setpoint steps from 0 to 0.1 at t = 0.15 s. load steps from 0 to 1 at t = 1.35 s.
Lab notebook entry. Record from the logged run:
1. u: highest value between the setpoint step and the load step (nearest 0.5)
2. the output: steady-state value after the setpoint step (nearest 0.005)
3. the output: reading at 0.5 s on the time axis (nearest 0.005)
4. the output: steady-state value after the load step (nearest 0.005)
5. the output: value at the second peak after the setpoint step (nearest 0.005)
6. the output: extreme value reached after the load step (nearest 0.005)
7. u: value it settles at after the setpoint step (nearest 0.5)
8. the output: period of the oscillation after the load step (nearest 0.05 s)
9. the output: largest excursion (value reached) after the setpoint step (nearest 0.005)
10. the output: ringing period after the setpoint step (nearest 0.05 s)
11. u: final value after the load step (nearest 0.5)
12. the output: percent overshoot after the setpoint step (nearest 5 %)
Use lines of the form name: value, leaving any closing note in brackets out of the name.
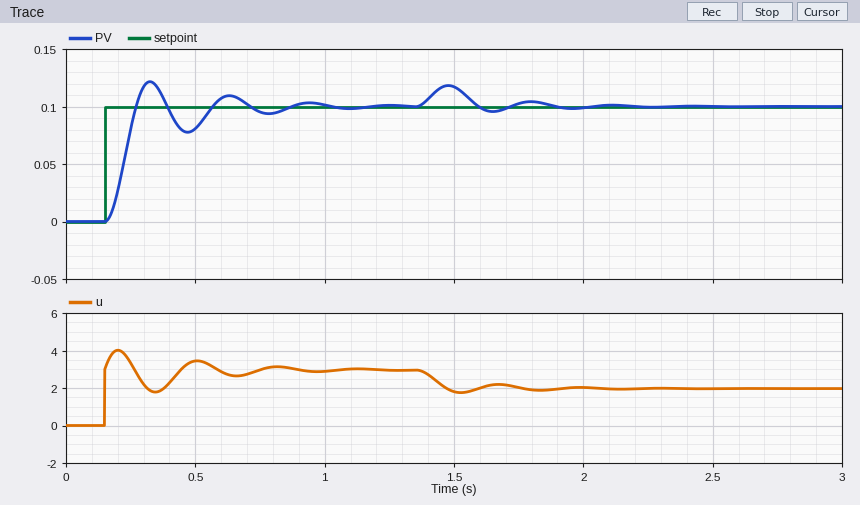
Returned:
u: highest value between the setpoint step and the load step: 4.0
the output: steady-state value after the setpoint step: 0.100
the output: reading at 0.5 s on the time axis: 0.080
the output: steady-state value after the load step: 0.100
the output: value at the second peak after the setpoint step: 0.110
the output: extreme value reached after the load step: 0.120
u: value it settles at after the setpoint step: 3.0
the output: period of the oscillation after the load step: 0.30 s
the output: largest excursion (value reached) after the setpoint step: 0.120
the output: ringing period after the setpoint step: 0.30 s
u: final value after the load step: 2.0
the output: percent overshoot after the setpoint step: 20 %
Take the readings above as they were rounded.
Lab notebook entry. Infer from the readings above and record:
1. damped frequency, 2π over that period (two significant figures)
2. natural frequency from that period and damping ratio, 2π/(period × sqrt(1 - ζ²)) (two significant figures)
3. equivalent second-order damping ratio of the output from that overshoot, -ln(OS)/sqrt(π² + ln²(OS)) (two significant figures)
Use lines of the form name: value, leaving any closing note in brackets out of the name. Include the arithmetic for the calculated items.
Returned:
damped frequency, 2π over that period: 2π / 0.3 = 21 rad/s
natural frequency from that period and damping ratio, 2π/(period × sqrt(1 - ζ²)): 2π / (0.3 × sqrt(1 - 0.46²)) = 24 rad/s
equivalent second-order damping ratio of the output from that overshoot, -ln(OS)/sqrt(π² + ln²(OS)): ln(0.2) = -1.609; 1.609 / sqrt(9.870 + 2.590) = 0.46
